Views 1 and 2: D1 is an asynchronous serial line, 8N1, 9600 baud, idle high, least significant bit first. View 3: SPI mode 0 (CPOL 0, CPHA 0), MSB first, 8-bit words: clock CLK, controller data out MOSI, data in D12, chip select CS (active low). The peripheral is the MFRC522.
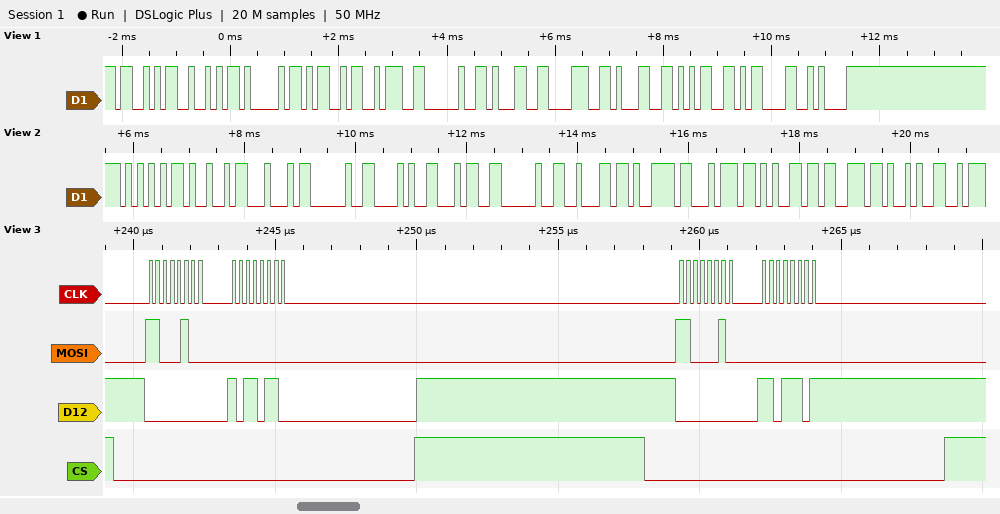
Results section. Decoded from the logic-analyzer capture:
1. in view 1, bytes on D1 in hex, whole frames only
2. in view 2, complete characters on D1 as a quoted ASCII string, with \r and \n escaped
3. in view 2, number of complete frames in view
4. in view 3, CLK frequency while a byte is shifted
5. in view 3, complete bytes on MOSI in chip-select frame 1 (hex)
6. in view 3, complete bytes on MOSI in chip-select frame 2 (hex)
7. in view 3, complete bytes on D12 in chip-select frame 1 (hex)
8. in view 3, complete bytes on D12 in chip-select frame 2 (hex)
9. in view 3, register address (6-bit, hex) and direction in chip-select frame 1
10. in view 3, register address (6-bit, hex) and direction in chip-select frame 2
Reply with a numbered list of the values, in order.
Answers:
1. 53 52 41 4D 3A 20 31 38 31 35 0D 0A
2. "UID (4 bytes)"
3. 13
4. 4 MHz
5. C4 00
6. C2 00
7. 00 B6
8. 00 DD
9. 0x22 read
10. 0x21 read
